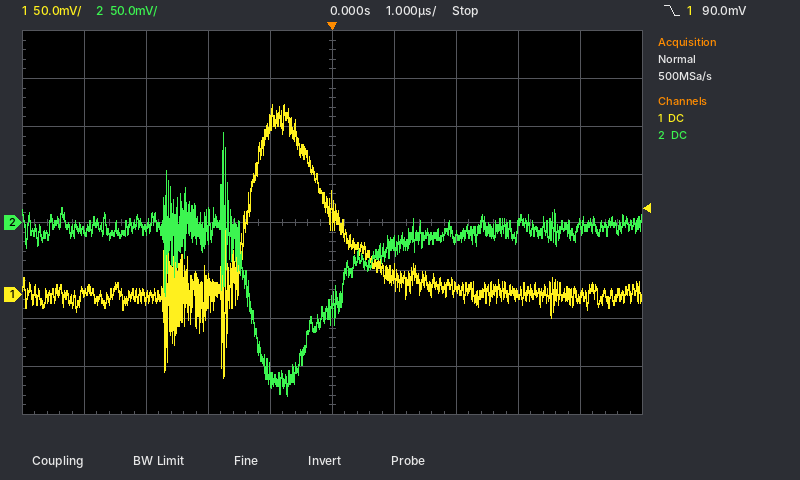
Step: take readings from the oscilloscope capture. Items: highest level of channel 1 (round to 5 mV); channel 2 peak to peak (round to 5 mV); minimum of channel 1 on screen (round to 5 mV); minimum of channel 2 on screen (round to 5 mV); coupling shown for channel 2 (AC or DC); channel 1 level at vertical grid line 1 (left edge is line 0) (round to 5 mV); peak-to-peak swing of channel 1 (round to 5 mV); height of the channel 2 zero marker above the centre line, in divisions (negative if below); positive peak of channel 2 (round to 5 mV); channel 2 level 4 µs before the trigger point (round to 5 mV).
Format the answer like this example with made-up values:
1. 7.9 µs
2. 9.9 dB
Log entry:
1. 200 mV
2. 275 mV
3. -85 mV
4. -180 mV
5. DC
6. 5 mV
7. 285 mV
8. 0.0 div
9. 95 mV
10. -10 mV
